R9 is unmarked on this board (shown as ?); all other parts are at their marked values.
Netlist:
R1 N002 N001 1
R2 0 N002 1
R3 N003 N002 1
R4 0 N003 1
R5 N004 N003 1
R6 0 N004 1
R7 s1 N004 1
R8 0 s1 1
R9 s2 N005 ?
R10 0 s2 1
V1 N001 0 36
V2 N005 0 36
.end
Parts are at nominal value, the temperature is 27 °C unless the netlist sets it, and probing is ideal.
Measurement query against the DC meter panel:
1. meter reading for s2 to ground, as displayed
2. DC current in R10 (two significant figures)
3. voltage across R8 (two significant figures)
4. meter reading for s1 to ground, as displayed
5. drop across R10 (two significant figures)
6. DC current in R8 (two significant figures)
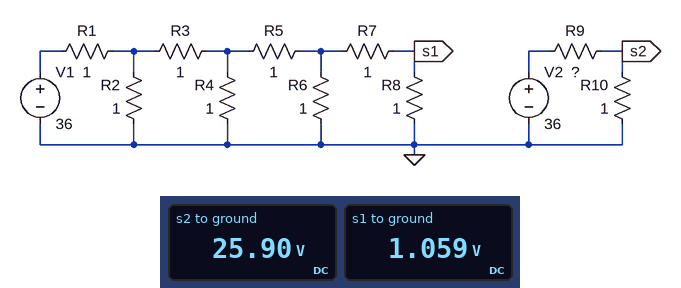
25.90 V
26 A
1.1 V
1.059 V
26 V
1.1 A
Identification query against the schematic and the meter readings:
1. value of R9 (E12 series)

0.39 Ω
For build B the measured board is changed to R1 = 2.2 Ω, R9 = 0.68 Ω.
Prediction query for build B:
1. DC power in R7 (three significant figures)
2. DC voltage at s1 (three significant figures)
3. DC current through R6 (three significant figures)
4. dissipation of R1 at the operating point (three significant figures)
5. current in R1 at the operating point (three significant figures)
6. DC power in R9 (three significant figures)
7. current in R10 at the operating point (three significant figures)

370 mW
608 mV
1.22 A
359 W
12.8 A
312 W
21.4 A
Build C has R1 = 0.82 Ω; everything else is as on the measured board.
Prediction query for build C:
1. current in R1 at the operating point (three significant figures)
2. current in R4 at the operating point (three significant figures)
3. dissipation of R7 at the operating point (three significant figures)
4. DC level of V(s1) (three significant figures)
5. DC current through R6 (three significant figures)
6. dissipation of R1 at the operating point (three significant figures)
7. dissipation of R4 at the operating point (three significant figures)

25.0 A
5.96 A
1.42 W
1.19 V
2.38 A
513 W
35.5 W
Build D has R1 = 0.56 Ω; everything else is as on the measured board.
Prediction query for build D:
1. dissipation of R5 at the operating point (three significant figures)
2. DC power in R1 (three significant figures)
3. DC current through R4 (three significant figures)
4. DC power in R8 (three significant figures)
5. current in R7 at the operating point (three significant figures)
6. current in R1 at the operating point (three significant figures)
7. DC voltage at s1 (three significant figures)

19.0 W
522 W
7.27 A
2.11 W
1.45 A
30.5 A
1.45 V
